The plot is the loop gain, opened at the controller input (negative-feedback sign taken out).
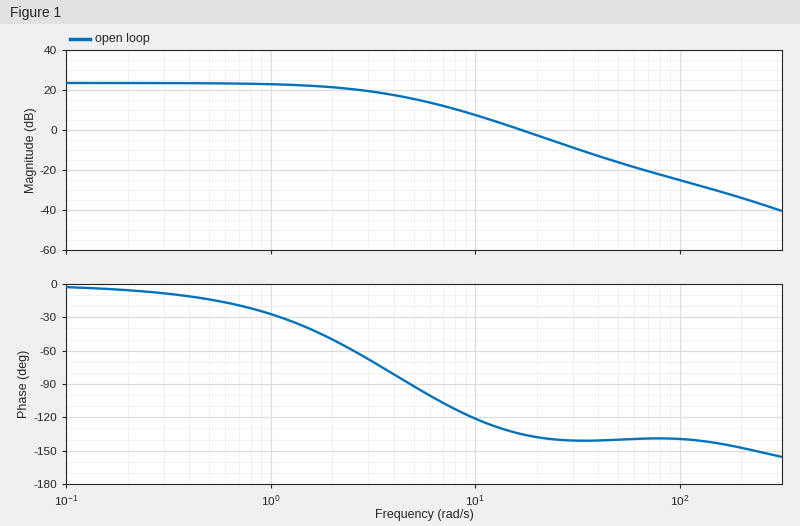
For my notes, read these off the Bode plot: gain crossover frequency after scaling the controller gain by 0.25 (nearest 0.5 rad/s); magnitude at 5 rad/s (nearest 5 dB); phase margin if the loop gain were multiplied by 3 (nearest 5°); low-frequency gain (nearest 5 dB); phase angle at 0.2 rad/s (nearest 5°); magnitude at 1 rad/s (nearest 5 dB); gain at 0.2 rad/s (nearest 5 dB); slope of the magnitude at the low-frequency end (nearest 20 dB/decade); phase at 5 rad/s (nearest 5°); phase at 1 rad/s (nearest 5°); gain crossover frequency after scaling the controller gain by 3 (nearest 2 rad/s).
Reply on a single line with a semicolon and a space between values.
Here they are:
7.0 rad/s; 15 dB; 40°; 25 dB; -5°; 25 dB; 25 dB; 0 dB/decade; -90°; -25°; 32 rad/s
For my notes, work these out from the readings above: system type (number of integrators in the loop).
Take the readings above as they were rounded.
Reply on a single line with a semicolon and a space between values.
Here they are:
0
